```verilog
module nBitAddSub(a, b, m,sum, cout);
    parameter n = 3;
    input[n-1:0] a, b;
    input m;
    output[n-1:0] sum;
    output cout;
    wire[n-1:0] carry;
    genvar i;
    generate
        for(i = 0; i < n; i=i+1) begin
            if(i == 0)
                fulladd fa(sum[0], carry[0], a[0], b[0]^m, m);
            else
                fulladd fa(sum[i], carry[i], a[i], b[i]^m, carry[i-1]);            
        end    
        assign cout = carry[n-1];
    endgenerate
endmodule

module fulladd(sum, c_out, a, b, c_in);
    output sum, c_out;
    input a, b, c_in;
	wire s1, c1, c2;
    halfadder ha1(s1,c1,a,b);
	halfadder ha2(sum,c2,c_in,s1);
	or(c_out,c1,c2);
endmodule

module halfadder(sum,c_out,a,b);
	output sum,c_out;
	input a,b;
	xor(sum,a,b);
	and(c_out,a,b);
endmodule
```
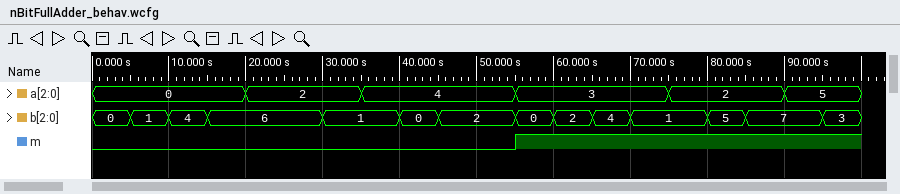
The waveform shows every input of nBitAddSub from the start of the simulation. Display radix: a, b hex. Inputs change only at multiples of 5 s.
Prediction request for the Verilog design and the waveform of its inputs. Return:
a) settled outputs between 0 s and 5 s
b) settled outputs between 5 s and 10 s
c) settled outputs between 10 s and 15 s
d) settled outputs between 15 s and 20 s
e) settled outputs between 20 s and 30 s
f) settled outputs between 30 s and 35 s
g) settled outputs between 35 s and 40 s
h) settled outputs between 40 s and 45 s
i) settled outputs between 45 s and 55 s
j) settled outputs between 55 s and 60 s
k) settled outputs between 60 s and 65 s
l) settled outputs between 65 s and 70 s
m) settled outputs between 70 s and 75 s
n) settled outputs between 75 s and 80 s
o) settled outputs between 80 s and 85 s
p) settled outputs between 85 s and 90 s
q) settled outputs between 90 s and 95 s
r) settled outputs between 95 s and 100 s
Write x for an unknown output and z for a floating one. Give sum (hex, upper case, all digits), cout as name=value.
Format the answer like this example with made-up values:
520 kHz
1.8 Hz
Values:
sum=0, cout=0
sum=1, cout=0
sum=4, cout=0
sum=6, cout=0
sum=0, cout=1
sum=3, cout=0
sum=5, cout=0
sum=4, cout=0
sum=6, cout=0
sum=3, cout=1
sum=1, cout=1
sum=7, cout=0
sum=2, cout=1
sum=1, cout=1
sum=5, cout=0
sum=3, cout=0
sum=6, cout=0
sum=2, cout=1
